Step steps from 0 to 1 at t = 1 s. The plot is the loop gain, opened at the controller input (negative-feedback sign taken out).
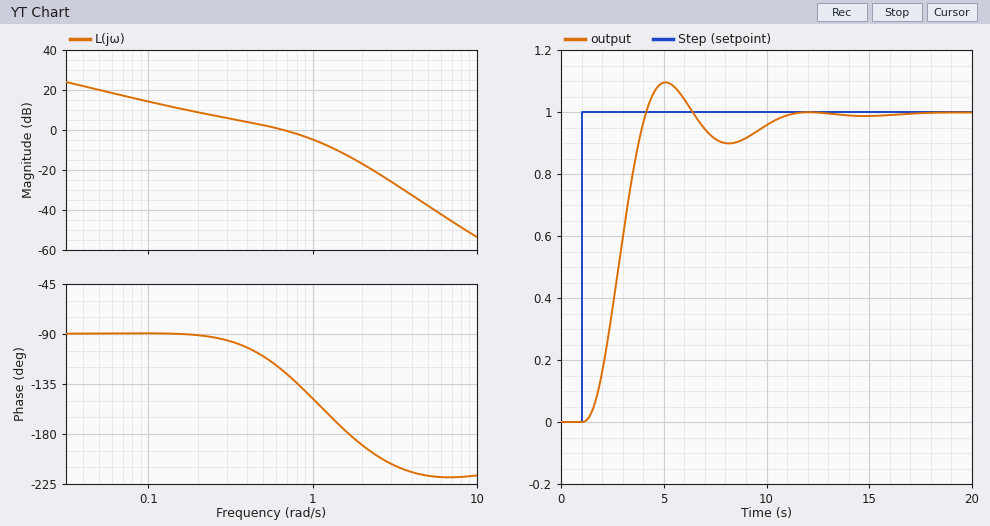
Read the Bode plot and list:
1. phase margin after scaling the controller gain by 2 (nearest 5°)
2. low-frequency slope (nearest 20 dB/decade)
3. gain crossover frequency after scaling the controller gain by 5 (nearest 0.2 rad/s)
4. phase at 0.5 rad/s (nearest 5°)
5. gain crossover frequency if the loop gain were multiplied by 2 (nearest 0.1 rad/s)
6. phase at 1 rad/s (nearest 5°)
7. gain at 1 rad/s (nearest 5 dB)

25°
-20 dB/decade
1.8 rad/s
-110°
1.1 rad/s
-150°
-5 dB
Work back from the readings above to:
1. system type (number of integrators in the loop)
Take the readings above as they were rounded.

1
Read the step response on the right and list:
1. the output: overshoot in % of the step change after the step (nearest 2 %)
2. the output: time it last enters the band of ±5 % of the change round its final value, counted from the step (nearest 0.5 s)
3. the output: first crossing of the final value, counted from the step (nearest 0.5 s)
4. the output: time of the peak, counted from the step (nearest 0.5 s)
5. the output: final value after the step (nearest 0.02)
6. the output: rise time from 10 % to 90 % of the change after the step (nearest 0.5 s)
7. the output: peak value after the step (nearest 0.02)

10 %
9.0 s
3.0 s
4.0 s
1.00
2.0 s
1.10
